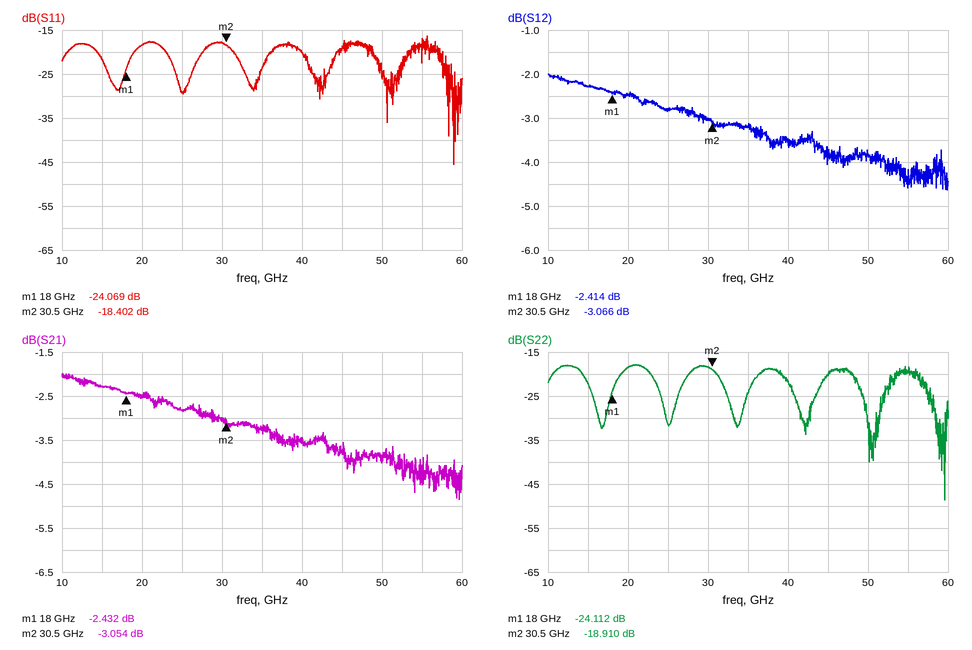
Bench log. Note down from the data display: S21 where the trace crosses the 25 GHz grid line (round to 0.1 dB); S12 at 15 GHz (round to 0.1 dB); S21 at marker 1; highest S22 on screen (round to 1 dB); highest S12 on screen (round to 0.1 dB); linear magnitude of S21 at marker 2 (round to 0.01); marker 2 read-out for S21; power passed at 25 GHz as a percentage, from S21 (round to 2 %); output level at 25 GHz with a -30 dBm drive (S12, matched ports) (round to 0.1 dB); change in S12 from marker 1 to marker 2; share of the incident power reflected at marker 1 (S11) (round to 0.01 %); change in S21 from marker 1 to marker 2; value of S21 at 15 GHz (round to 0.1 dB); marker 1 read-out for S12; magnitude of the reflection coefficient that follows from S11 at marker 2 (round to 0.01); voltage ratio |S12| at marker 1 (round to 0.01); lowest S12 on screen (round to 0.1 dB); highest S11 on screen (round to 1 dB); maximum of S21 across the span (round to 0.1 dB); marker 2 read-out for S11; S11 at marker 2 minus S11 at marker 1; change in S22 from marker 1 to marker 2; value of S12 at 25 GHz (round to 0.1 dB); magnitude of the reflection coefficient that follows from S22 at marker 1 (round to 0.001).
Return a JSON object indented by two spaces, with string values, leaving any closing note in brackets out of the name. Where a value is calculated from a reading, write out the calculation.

{
  "S21 where the trace crosses the 25 GHz grid line": "-2.8 dB",
  "S12 at 15 GHz": "-2.3 dB",
  "S21 at marker 1": "-2.432 dB",
  "highest S22 on screen": "-18 dB",
  "highest S12 on screen": "-2.0 dB",
  "linear magnitude of S21 at marker 2": "10^(-3.054/20) ≈ 0.70",
  "marker 2 read-out for S21": "-3.054 dB",
  "power passed at 25 GHz as a percentage, from S21": "10^(-2.8/10) ≈ 52 %",
  "output level at 25 GHz with a -30 dBm drive (S12, matched ports)": "-30 dBm + (-2.8 dB) = -32.8 dBm",
  "change in S12 from marker 1 to marker 2": "-3.066 − (-2.414) = -0.652 dB",
  "share of the incident power reflected at marker 1 (S11)": "10^(-24.069/10) ≈ 0.39 %",
  "change in S21 from marker 1 to marker 2": "-3.054 − (-2.432) = -0.622 dB",
  "value of S21 at 15 GHz": "-2.3 dB",
  "marker 1 read-out for S12": "-2.414 dB",
  "magnitude of the reflection coefficient that follows from S11 at marker 2": "10^(-18.402/20) ≈ 0.12",
  "voltage ratio |S12| at marker 1": "10^(-2.414/20) ≈ 0.76",
  "lowest S12 on screen": "-4.6 dB",
  "highest S11 on screen": "-16 dB",
  "maximum of S21 across the span": "-2.0 dB",
  "marker 2 read-out for S11": "-18.402 dB",
  "S11 at marker 2 minus S11 at marker 1": "-18.402 − (-24.069) = 5.667 dB",
  "change in S22 from marker 1 to marker 2": "-18.91 − (-24.112) = 5.202 dB",
  "value of S12 at 25 GHz": "-2.8 dB",
  "magnitude of the reflection coefficient that follows from S22 at marker 1": "10^(-24.112/20) ≈ 0.062"
}
